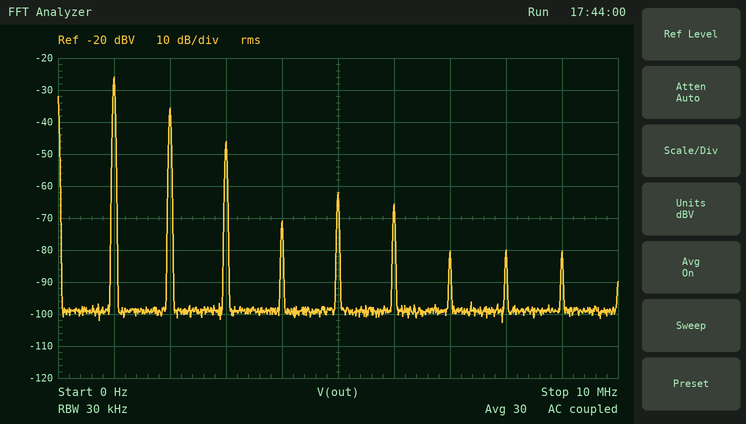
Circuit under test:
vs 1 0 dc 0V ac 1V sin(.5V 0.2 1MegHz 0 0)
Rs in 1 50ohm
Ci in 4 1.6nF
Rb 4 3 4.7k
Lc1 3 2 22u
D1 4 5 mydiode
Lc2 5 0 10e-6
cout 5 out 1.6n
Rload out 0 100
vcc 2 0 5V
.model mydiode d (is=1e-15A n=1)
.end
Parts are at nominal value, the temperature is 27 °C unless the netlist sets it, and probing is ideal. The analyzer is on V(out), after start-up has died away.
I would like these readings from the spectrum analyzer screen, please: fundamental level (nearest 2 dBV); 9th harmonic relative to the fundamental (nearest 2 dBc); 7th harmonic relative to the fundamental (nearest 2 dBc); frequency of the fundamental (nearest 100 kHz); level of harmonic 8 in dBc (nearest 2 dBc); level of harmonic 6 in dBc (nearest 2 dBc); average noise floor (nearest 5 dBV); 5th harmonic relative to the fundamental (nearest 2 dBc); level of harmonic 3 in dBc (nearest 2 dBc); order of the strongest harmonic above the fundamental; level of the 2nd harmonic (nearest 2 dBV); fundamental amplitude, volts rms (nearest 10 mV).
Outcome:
-26 dBV
-54 dBc
-54 dBc
1.0 MHz
-54 dBc
-40 dBc
-100 dBV
-36 dBc
-20 dBc
2
-36 dBV
50 mV
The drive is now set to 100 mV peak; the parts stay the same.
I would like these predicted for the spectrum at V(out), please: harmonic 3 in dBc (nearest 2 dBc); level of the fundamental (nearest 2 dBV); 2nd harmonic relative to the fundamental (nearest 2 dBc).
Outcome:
-34 dBc
-30 dBV
-22 dBc
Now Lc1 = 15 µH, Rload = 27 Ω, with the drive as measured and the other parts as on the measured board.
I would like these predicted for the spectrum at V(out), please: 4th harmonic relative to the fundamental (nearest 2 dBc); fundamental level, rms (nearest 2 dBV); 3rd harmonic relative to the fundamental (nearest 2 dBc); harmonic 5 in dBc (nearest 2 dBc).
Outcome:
-36 dBc
-30 dBV
-24 dBc
-40 dBc
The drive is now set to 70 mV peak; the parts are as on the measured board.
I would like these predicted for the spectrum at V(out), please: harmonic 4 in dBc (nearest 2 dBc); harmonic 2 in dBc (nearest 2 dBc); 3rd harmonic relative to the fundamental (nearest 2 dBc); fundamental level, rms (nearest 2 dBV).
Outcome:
-56 dBc
-26 dBc
-42 dBc
-32 dBV
